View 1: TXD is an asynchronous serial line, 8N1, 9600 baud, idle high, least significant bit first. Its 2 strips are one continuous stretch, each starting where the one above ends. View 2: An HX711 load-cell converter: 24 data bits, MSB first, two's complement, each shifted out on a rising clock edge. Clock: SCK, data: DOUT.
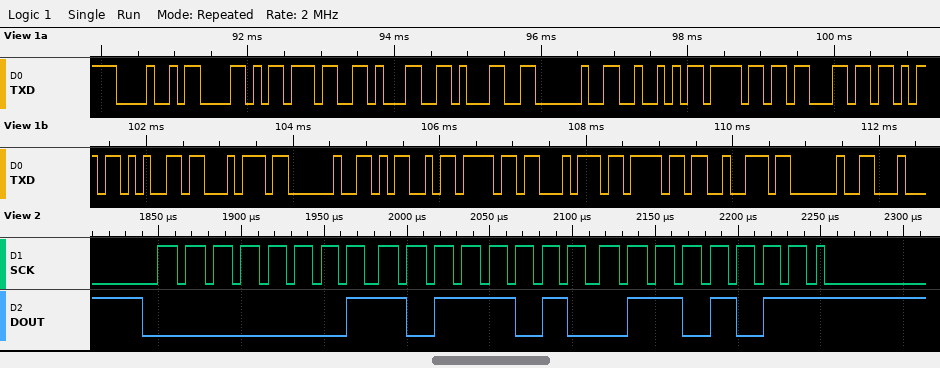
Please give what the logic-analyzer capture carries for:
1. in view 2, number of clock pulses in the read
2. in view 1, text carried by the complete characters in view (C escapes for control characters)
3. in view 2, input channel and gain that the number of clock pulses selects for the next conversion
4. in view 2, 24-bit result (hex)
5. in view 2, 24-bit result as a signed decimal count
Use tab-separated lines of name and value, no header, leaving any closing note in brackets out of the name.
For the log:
in view 2, number of clock pulses in the read	25
in view 1, text carried by the complete characters in view	"HX711 Rocket Motor "
in view 2, input channel and gain that the number of clock pulses selects for the next conversion	channel A, gain 128
in view 2, 24-bit result	0x01BA6B
in view 2, 24-bit result as a signed decimal count	113259
